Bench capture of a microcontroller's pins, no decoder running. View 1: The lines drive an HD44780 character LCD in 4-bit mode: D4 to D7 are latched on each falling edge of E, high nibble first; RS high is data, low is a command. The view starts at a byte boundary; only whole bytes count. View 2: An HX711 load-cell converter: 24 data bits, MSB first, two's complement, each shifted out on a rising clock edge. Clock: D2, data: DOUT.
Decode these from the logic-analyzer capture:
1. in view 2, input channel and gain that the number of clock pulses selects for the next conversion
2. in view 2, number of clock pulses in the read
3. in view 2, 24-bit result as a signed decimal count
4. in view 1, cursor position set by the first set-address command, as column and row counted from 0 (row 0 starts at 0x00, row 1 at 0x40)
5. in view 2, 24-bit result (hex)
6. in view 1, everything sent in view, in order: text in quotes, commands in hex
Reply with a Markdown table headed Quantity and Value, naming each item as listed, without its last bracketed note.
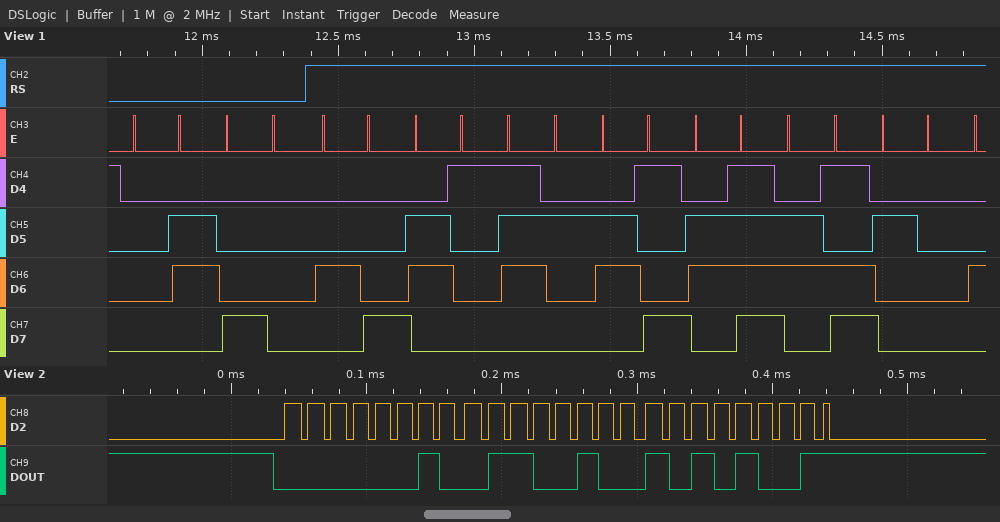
| Quantity | Value |
|---|---|
| in view 2, input channel and gain that the number of clock pulses selects for the next conversion | channel A, gain 128 |
| in view 2, number of clock pulses in the read | 25 |
| in view 2, 24-bit result as a signed decimal count | 156841 |
| in view 1, cursor position set by the first set-address command, as column and row counted from 0 | column 0, row 0 |
| in view 2, 24-bit result | 0x0264A9 |
| in view 1, everything sent in view, in order: text in quotes, commands in hex | 0x06 0x80 "Hariom " |
